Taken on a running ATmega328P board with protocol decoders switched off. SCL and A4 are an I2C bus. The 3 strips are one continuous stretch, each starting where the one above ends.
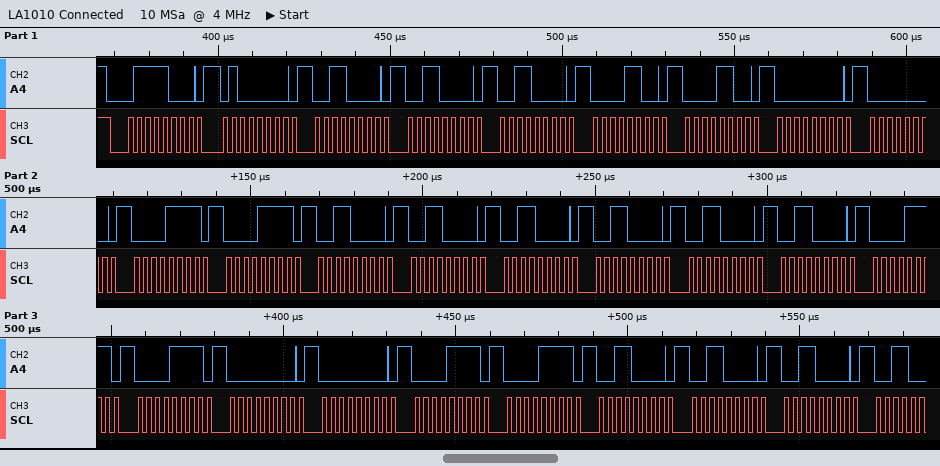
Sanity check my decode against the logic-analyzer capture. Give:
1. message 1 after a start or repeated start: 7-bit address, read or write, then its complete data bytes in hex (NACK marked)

0x3C write: 40 30 30 30 0C 0C 00 00 0F 0F 30 30 30 30 30 30 0F 0F 00 00 0F 0F 30 30 30
